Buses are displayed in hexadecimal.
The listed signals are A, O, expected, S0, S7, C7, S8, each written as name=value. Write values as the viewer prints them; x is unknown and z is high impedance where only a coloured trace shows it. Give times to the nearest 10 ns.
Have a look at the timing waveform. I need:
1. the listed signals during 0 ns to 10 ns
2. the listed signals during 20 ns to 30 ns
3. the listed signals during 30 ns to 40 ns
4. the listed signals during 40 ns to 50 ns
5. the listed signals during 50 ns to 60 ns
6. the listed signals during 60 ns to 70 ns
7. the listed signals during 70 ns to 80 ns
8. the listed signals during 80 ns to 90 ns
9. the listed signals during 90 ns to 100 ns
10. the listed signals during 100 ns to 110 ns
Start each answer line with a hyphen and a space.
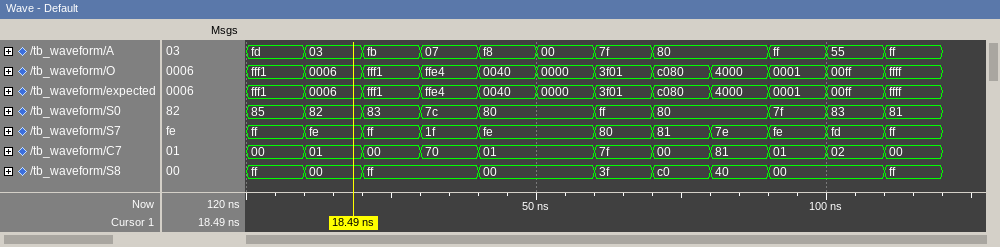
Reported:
- A=fd, O=fff1, expected=fff1, S0=85, S7=ff, C7=00, S8=ff
- A=fb, O=fff1, expected=fff1, S0=83, S7=ff, C7=00, S8=ff
- A=07, O=ffe4, expected=ffe4, S0=7c, S7=1f, C7=70, S8=ff
- A=f8, O=0040, expected=0040, S0=80, S7=fe, C7=01, S8=00
- A=00, O=0000, expected=0000, S0=80, S7=fe, C7=01, S8=00
- A=7f, O=3f01, expected=3f01, S0=ff, S7=80, C7=7f, S8=3f
- A=80, O=c080, expected=c080, S0=80, S7=81, C7=00, S8=c0
- A=80, O=4000, expected=4000, S0=80, S7=7e, C7=81, S8=40
- A=ff, O=0001, expected=0001, S0=7f, S7=fe, C7=01, S8=00
- A=55, O=00ff, expected=00ff, S0=83, S7=fd, C7=02, S8=00
